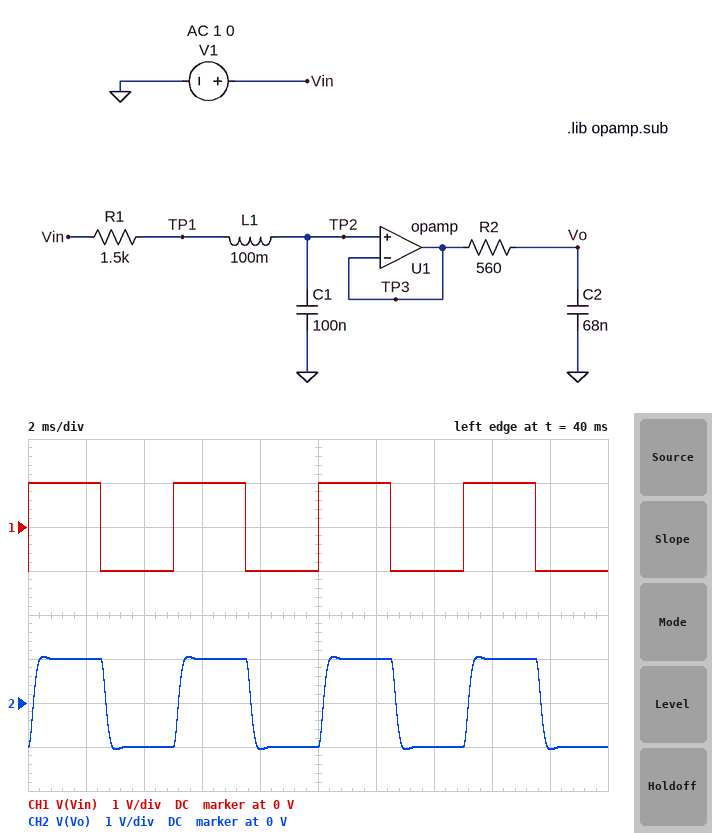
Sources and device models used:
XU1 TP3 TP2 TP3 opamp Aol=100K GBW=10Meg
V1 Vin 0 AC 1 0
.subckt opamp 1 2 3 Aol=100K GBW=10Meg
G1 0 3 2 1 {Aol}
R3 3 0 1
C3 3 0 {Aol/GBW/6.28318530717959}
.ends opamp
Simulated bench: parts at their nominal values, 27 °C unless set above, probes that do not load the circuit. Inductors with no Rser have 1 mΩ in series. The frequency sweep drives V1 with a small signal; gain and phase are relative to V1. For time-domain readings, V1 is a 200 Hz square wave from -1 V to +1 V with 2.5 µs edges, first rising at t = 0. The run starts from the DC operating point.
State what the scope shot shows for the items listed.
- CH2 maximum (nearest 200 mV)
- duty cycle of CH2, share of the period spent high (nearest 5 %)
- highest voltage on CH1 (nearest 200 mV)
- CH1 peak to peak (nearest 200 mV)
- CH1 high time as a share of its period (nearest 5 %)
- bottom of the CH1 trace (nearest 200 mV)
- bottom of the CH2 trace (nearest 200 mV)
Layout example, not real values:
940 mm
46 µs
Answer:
1.0 V
50 %
1.0 V
2.0 V
50 %
-1.0 V
-1.0 V
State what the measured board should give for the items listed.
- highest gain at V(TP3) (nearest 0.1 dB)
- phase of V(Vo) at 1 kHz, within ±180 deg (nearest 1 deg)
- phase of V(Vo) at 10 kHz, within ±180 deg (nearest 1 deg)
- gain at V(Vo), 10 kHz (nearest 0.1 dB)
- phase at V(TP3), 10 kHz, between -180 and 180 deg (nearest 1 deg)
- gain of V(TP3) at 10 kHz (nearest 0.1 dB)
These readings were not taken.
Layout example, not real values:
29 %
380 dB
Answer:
0 dB
-71 deg
126 deg
-40.2 dB
-166 deg
-32.0 dB
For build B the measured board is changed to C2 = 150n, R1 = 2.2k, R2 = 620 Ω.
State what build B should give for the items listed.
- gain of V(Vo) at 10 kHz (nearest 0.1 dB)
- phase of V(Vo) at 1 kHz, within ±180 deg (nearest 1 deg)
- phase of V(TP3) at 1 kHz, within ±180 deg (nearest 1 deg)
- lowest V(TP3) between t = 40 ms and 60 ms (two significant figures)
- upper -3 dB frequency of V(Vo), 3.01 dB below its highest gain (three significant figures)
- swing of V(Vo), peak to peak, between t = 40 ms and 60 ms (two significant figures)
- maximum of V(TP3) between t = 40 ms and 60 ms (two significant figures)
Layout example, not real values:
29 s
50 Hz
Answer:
-47.7 dB
-97 deg
-66 deg
-1.0 V
749 Hz
2.0 V
1.0 V
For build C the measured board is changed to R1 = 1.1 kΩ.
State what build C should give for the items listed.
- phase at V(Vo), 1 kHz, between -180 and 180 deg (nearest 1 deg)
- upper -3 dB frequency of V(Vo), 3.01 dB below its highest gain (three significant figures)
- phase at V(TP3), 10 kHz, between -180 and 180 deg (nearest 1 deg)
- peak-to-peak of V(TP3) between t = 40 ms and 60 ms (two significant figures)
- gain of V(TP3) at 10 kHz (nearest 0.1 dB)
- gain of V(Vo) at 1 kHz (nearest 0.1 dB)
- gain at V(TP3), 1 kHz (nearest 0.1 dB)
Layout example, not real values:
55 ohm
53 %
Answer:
-62 deg
1.75 kHz
-170 deg
2.5 V
-31.8 dB
0.5 dB
0.7 dB
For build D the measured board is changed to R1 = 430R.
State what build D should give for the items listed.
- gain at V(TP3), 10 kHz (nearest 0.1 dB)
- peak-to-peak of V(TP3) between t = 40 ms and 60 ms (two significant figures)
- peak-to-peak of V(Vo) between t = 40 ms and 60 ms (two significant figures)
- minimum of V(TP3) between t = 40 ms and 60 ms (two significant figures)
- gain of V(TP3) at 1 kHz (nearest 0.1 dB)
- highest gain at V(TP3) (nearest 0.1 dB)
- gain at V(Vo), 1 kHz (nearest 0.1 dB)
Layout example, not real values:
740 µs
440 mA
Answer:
-31.7 dB
4.0 V
3.9 V
-2.0 V
3.6 dB
7.5 dB
3.3 dB
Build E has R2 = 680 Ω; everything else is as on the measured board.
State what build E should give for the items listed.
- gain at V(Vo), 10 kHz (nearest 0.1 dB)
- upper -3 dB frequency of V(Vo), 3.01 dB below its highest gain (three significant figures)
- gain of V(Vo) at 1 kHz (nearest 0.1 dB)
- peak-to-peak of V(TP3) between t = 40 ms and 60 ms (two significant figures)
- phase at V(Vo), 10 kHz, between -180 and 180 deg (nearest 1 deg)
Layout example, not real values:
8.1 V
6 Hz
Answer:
-41.7 dB
1.37 kHz
-1.3 dB
2.1 V
123 deg
